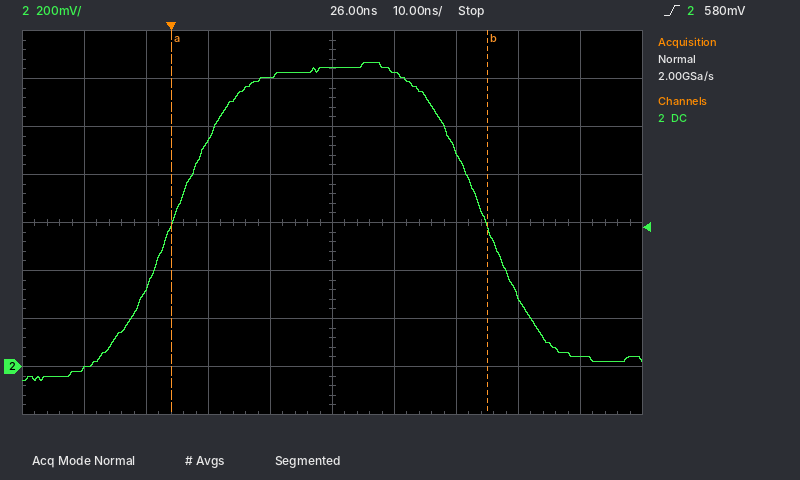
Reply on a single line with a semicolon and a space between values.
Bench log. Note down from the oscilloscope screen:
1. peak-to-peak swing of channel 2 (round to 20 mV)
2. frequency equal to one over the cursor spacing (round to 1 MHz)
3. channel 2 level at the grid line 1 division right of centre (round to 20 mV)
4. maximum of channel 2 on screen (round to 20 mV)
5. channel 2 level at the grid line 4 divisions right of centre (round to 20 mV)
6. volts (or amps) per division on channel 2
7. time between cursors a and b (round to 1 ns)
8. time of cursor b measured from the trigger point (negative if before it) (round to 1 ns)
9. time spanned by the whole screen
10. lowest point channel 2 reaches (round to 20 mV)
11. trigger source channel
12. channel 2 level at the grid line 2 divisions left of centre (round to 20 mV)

1.32 V; 20 MHz; 1.22 V; 1.26 V; 40 mV; 200 mV; 51 ns; +51 ns; 100 ns; -60 mV; channel 2; 940 mV
